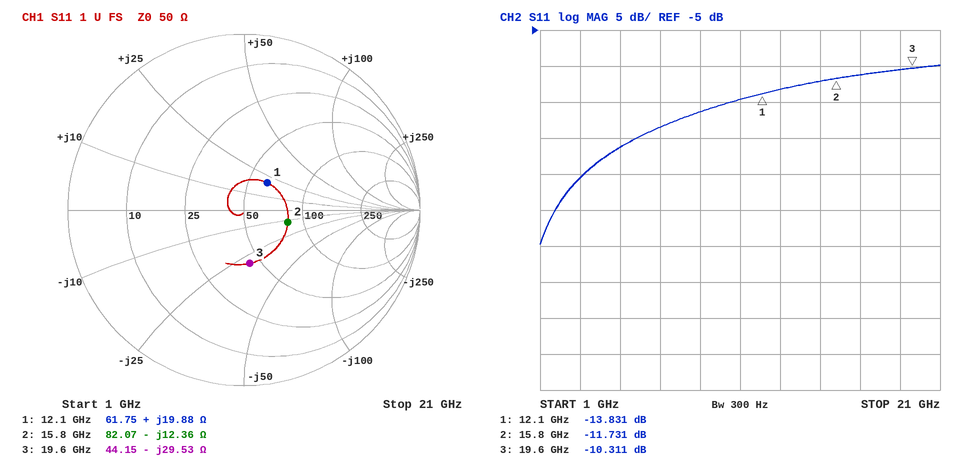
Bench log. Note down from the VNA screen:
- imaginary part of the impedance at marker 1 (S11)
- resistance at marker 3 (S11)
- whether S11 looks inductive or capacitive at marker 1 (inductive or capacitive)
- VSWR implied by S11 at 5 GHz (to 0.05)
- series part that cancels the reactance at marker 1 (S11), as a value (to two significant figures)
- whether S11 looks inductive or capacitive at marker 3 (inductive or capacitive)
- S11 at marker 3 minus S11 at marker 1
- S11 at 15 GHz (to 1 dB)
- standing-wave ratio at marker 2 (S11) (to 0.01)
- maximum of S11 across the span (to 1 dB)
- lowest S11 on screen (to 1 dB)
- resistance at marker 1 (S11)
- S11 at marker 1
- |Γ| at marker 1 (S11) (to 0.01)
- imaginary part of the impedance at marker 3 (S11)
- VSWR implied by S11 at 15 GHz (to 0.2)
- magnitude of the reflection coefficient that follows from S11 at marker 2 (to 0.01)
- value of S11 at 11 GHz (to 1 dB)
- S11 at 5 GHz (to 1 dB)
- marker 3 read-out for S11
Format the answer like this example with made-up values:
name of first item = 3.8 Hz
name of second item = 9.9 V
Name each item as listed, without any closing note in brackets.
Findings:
imaginary part of the impedance at marker 1 = +19.88 Ω
resistance at marker 3 = 44.15 Ω
whether S11 looks inductive or capacitive at marker 1 = inductive
VSWR implied by S11 at 5 GHz = 1.20
series part that cancels the reactance at marker 1 (S11), as a value = 660 fF
whether S11 looks inductive or capacitive at marker 3 = capacitive
S11 at marker 3 minus S11 at marker 1 = 3.520 dB
S11 at 15 GHz = -12 dB
standing-wave ratio at marker 2 (S11) = 1.70
maximum of S11 across the span = -10 dB
lowest S11 on screen = -35 dB
resistance at marker 1 = 61.75 Ω
S11 at marker 1 = -13.831 dB
|Γ| at marker 1 (S11) = 0.20
imaginary part of the impedance at marker 3 = -29.53 Ω
VSWR implied by S11 at 15 GHz = 1.6
magnitude of the reflection coefficient that follows from S11 at marker 2 = 0.26
value of S11 at 11 GHz = -15 dB
S11 at 5 GHz = -21 dB
marker 3 read-out for S11 = -10.311 dB
